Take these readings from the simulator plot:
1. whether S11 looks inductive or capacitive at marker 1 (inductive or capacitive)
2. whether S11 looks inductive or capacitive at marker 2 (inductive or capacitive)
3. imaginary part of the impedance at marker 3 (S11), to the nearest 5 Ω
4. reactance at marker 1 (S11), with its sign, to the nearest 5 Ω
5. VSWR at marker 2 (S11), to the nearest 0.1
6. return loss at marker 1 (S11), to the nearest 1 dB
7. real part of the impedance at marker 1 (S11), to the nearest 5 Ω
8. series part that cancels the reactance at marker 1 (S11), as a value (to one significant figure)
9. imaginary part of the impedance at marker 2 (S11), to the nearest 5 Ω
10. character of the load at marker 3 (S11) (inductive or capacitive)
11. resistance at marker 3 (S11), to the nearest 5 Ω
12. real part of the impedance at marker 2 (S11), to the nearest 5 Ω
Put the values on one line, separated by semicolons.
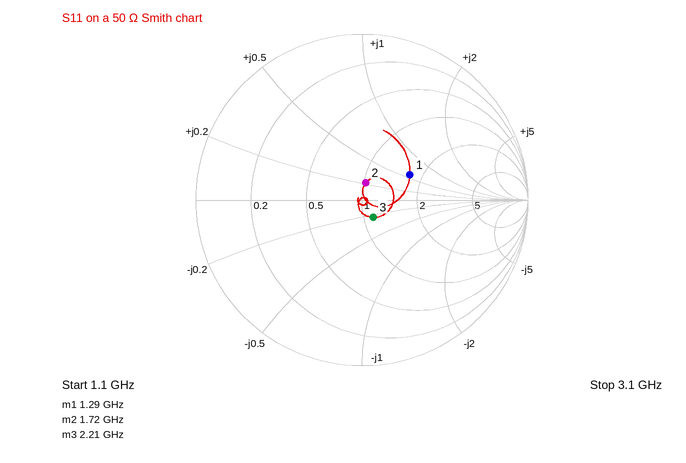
inductive; inductive; -10 Ω; +30 Ω; 1.2; 10 dB; 85 Ω; 4 pF; +10 Ω; capacitive; 55 Ω; 50 Ω
